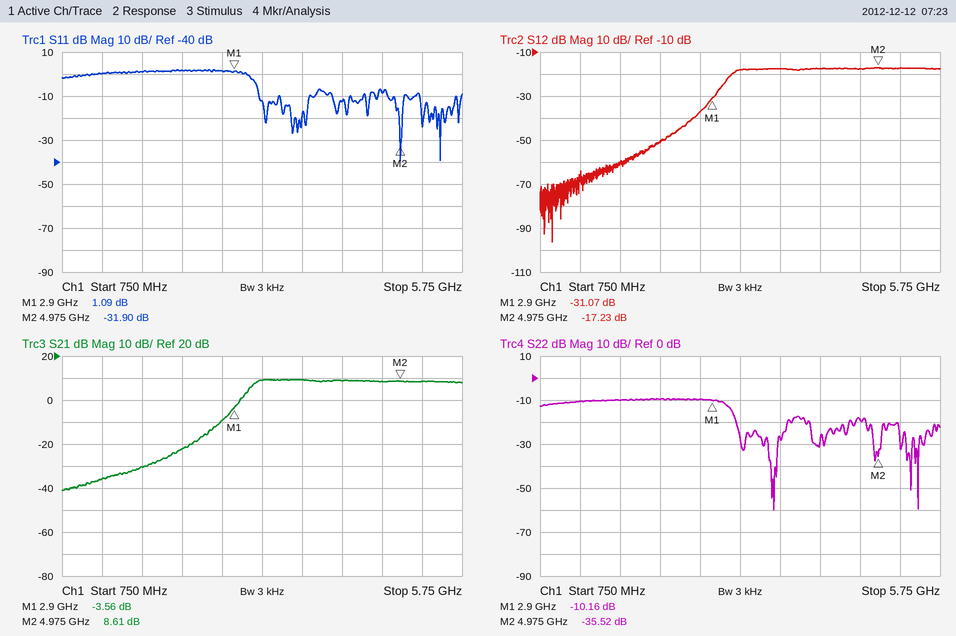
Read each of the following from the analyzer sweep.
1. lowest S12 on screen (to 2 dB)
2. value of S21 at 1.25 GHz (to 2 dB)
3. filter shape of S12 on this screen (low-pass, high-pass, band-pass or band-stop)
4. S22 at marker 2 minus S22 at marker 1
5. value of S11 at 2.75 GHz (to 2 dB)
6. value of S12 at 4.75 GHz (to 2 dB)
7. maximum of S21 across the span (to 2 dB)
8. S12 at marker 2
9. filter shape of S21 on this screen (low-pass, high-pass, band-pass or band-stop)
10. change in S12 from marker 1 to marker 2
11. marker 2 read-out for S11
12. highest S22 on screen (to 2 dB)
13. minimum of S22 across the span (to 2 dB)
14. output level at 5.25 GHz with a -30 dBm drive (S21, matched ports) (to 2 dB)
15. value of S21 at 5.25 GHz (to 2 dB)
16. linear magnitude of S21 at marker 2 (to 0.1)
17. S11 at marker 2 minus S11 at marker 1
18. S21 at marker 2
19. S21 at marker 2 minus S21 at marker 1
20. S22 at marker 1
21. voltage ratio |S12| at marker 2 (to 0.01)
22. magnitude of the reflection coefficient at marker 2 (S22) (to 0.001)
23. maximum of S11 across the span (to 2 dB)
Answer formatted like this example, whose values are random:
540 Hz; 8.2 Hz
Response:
-96 dB; -36 dB; high-pass; -25.36 dB; 2 dB; -18 dB; 10 dB; -17.23 dB; high-pass; 13.84 dB; -31.90 dB; -10 dB; -60 dB; -22 dBm; 8 dB; 2.7; -32.99 dB; 8.61 dB; 12.17 dB; -10.16 dB; 0.14; 0.017; 2 dB
